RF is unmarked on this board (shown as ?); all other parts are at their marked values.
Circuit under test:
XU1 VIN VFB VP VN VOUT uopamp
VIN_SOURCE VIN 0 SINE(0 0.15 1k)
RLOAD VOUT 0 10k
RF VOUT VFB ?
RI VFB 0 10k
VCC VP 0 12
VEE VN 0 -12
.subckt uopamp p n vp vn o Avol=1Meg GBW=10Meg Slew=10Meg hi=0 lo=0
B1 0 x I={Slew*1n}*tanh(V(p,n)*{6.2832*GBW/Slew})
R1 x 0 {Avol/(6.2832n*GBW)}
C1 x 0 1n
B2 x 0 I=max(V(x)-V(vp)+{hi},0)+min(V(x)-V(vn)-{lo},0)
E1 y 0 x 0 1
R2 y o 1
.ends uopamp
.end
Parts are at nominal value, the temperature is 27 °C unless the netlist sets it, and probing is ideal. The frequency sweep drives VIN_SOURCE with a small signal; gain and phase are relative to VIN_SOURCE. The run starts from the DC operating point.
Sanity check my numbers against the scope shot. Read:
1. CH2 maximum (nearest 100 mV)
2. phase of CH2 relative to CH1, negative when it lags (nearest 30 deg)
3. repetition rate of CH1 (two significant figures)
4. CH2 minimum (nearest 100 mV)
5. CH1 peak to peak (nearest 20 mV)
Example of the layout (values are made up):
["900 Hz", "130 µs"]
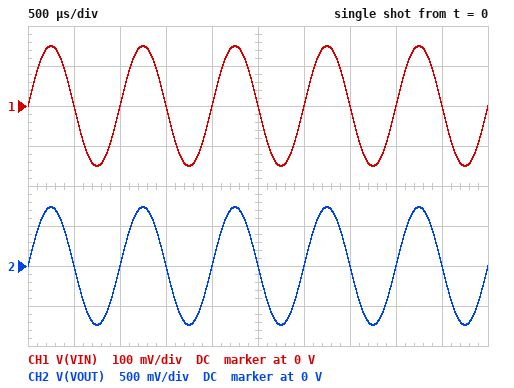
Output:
["700 mV", "0 deg", "1.0 kHz", "-700 mV", "300 mV"]
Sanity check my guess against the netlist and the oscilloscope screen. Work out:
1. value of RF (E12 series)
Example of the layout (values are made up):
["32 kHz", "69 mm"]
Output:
["39 kΩ"]
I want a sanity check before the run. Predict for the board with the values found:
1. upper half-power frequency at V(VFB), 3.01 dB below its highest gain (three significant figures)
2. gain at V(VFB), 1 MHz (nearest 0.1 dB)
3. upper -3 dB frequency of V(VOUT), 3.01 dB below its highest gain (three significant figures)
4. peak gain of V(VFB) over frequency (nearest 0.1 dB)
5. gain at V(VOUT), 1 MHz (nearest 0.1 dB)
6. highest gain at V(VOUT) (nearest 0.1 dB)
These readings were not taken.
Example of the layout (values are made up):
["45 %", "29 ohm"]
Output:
["2.04 MHz", "-0.9 dB", "2.04 MHz", "0 dB", "12.9 dB", "13.8 dB"]
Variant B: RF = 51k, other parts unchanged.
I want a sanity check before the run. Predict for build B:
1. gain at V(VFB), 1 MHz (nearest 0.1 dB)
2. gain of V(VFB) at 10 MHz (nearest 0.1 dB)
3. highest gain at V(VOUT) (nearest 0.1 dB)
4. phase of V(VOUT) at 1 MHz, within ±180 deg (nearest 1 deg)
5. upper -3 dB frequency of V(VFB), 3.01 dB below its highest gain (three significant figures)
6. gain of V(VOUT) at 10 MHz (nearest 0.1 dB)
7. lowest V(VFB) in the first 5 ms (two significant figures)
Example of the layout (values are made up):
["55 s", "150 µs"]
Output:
["-1.4 dB", "-15.8 dB", "15.7 dB", "-31 deg", "1.64 MHz", "-0.1 dB", "-150 mV"]
